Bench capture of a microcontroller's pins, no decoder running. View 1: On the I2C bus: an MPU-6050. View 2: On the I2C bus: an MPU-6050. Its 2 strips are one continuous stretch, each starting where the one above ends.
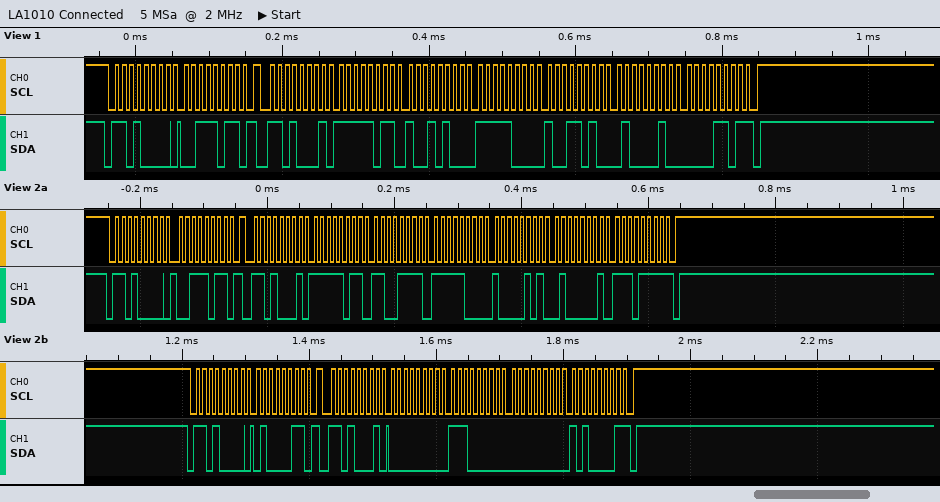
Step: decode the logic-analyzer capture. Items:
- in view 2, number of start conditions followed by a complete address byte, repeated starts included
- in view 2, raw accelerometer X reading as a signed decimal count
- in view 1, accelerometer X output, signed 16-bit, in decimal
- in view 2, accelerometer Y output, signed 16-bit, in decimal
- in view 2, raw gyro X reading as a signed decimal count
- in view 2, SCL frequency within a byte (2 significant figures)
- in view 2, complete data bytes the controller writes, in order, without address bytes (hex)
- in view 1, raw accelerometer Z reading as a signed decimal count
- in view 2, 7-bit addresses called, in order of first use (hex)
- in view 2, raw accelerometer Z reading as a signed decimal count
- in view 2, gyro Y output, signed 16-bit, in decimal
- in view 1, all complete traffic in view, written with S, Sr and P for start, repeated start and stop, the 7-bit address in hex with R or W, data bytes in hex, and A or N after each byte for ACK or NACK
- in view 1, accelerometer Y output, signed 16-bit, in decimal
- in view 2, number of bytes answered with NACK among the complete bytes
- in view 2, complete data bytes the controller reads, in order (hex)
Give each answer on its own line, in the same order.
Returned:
4
-1073
-1132
-1915
224
100 kHz
3B 43
16909
0x68
16879
161
S 68W A 3B A Sr 68R A FB A 94 A F8 A 9A A 42 A 0D N P
-1894
2
FB CF F8 85 41 EF 00 E0 00 A1
